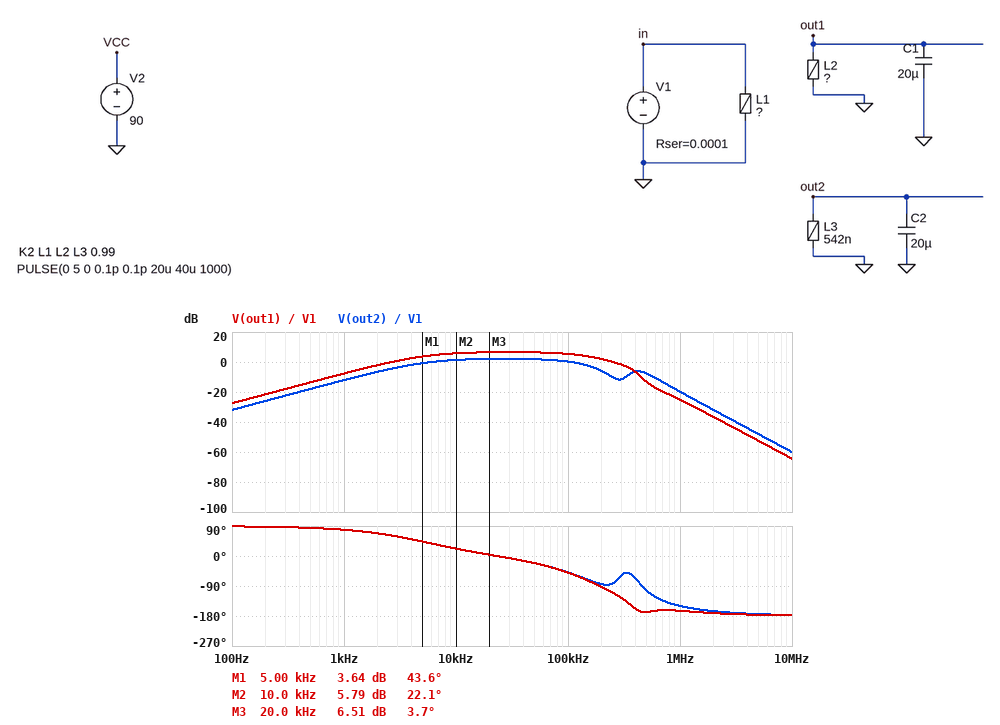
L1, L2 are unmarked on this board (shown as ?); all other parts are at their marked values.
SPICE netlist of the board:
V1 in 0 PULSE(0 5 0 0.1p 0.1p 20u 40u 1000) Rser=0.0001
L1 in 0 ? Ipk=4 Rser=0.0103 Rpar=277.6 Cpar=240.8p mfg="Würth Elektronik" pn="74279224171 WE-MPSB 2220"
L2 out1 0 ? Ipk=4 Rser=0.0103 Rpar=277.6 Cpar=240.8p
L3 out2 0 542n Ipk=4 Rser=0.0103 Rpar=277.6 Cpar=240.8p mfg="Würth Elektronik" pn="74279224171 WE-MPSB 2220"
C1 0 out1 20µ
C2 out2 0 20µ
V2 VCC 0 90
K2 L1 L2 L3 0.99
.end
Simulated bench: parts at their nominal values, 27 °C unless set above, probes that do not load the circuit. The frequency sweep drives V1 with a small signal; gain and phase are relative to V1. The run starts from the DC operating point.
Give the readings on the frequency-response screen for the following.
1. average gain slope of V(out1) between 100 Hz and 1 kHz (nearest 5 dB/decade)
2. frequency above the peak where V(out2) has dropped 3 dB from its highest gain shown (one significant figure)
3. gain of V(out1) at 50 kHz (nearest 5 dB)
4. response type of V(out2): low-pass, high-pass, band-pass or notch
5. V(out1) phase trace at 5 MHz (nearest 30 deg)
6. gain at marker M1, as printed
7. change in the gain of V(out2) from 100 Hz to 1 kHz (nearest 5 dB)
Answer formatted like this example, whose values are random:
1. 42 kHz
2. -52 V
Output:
1. 20 dB/decade
2. 100 kHz
3. 5 dB
4. band-pass
5. -180 deg
6. 3.64 dB
7. 20 dB
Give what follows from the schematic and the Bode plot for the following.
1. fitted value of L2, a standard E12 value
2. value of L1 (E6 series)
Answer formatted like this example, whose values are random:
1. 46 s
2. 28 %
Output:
1. 1.5 µH
2. 330 nH
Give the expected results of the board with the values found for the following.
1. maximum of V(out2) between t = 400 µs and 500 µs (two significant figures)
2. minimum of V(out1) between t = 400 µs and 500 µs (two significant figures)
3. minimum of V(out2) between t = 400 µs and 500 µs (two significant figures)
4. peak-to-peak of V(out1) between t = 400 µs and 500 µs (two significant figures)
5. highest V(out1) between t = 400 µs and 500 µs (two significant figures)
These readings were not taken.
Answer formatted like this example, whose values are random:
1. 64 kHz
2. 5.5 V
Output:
1. 3.9 V
2. -6.5 V
3. -3.9 V
4. 13 V
5. 6.5 V
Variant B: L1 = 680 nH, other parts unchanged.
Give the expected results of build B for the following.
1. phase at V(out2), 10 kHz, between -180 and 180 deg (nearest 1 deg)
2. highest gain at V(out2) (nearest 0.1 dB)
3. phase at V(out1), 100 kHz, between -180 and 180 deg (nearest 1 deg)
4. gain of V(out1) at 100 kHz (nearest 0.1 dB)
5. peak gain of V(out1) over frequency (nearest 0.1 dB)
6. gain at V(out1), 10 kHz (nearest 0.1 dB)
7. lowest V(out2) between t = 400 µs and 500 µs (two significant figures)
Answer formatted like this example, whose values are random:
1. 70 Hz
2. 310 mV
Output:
1. 11 deg
2. -0.6 dB
3. -34 deg
4. 4.5 dB
5. 5.0 dB
6. 3.2 dB
7. -3.1 V
